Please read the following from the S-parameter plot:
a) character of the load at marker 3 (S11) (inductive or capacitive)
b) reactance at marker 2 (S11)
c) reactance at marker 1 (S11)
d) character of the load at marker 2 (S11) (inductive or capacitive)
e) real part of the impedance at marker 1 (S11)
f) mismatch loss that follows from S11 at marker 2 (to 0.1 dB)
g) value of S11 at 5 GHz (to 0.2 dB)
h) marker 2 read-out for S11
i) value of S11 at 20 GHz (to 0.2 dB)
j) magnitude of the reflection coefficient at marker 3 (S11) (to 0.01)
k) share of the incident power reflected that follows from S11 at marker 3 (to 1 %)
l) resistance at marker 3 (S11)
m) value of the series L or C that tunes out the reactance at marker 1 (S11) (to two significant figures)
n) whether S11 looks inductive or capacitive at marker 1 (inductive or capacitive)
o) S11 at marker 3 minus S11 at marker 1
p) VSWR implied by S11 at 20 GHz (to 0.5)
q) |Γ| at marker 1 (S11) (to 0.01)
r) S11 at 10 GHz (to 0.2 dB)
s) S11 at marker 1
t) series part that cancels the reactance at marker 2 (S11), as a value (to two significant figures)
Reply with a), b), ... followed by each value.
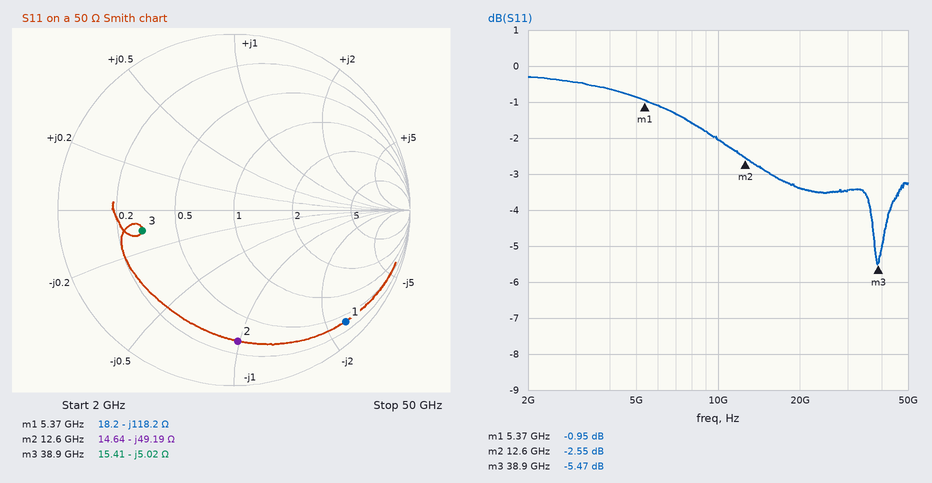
a) capacitive
b) -49.19 Ω
c) -118.2 Ω
d) capacitive
e) 18.2 Ω
f) 3.5 dB
g) -0.8 dB
h) -2.55 dB
i) -3.4 dB
j) 0.53
k) 28 %
l) 15.41 Ω
m) 3.5 nH
n) capacitive
o) -4.52 dB
p) 5.0
q) 0.90
r) -2.0 dB
s) -0.95 dB
t) 620 pH
